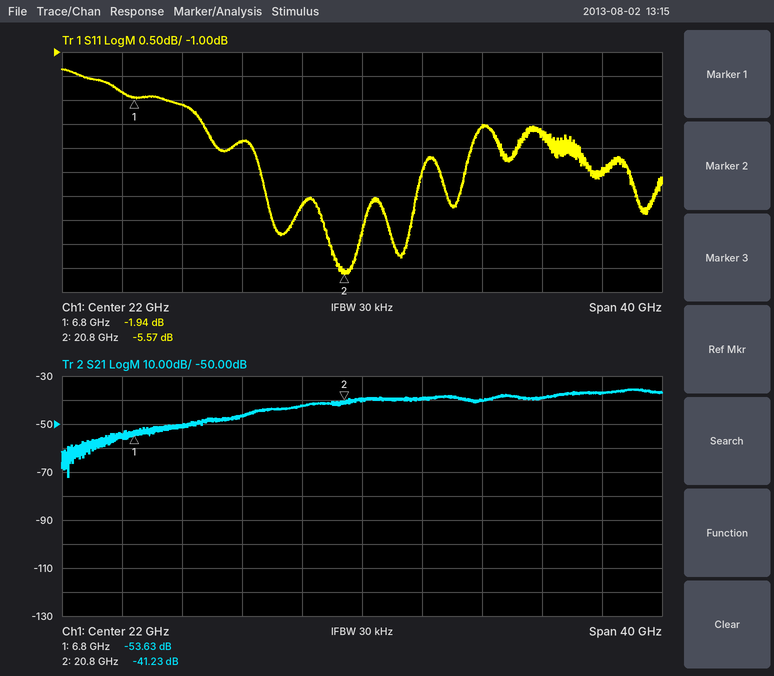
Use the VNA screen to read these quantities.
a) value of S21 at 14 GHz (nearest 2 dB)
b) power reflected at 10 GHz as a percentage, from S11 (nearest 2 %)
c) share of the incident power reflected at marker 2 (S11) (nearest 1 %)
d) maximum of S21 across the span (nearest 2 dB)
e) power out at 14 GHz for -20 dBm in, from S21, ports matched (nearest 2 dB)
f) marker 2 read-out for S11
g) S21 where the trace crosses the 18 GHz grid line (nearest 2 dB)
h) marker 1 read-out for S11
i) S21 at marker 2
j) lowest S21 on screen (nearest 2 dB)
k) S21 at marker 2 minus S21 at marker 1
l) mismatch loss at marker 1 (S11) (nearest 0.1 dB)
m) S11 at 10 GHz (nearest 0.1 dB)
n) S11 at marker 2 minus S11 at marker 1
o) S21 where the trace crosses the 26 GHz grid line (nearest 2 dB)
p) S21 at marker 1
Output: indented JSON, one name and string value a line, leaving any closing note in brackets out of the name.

{
  "value of S21 at 14 GHz": "-46 dB",
  "power reflected at 10 GHz as a percentage, from S11": "62 %",
  "share of the incident power reflected at marker 2 (S11)": "28 %",
  "maximum of S21 across the span": "-36 dB",
  "power out at 14 GHz for -20 dBm in, from S21, ports matched": "-66 dBm",
  "marker 2 read-out for S11": "-5.57 dB",
  "S21 where the trace crosses the 18 GHz grid line": "-42 dB",
  "marker 1 read-out for S11": "-1.94 dB",
  "S21 at marker 2": "-41.23 dB",
  "lowest S21 on screen": "-72 dB",
  "S21 at marker 2 minus S21 at marker 1": "12.40 dB",
  "mismatch loss at marker 1 (S11)": "4.4 dB",
  "S11 at 10 GHz": "-2.1 dB",
  "S11 at marker 2 minus S11 at marker 1": "-3.63 dB",
  "S21 where the trace crosses the 26 GHz grid line": "-40 dB",
  "S21 at marker 1": "-53.63 dB"
}
